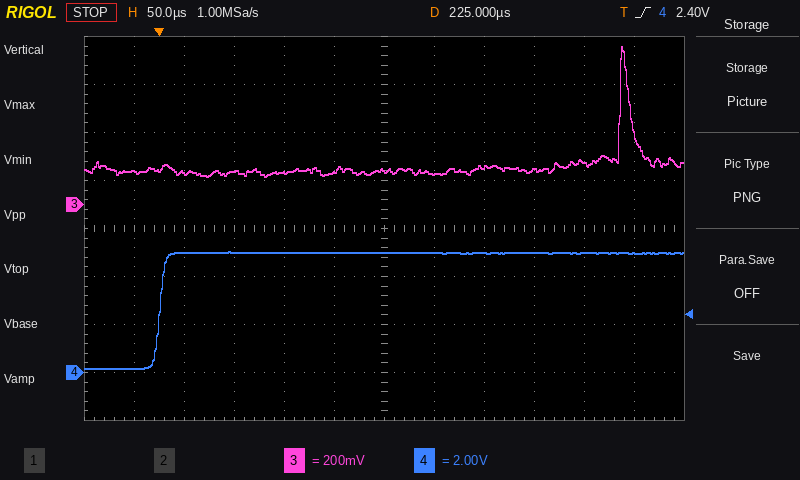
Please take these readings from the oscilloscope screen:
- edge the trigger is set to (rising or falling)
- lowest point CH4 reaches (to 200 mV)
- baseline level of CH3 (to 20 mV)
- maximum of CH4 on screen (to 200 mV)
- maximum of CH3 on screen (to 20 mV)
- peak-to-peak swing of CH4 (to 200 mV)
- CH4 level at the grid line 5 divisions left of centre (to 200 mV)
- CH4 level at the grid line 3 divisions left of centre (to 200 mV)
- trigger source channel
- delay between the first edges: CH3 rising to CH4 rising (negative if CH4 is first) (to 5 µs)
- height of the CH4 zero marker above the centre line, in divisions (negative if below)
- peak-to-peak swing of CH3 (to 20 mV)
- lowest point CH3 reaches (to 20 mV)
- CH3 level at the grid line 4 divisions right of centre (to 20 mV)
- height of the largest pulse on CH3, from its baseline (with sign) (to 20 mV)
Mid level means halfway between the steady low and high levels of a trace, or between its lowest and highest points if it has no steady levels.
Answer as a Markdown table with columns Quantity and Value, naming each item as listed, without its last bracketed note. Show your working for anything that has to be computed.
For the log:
| Quantity | Value |
|---|---|
| edge the trigger is set to | rising |
| lowest point CH4 reaches | 200 mV |
| baseline level of CH3 | 140 mV |
| maximum of CH4 on screen | 5.0 V |
| maximum of CH3 on screen | 660 mV |
| peak-to-peak swing of CH4 | 5.0 V − (200 mV) = 4.8 V |
| CH4 level at the grid line 5 divisions left of centre | 200 mV |
| CH4 level at the grid line 3 divisions left of centre | 5.0 V |
| trigger source channel | CH4 |
| delay between the first edges: CH3 rising to CH4 rising (negative if CH4 is first) | -460 µs |
| height of the CH4 zero marker above the centre line, in divisions | -3.0 div |
| peak-to-peak swing of CH3 | 660 mV − (120 mV) = 540 mV |
| lowest point CH3 reaches | 120 mV |
| CH3 level at the grid line 4 divisions right of centre | 180 mV |
| height of the largest pulse on CH3, from its baseline (with sign) | 660 mV − (140 mV) = +520 mV |
